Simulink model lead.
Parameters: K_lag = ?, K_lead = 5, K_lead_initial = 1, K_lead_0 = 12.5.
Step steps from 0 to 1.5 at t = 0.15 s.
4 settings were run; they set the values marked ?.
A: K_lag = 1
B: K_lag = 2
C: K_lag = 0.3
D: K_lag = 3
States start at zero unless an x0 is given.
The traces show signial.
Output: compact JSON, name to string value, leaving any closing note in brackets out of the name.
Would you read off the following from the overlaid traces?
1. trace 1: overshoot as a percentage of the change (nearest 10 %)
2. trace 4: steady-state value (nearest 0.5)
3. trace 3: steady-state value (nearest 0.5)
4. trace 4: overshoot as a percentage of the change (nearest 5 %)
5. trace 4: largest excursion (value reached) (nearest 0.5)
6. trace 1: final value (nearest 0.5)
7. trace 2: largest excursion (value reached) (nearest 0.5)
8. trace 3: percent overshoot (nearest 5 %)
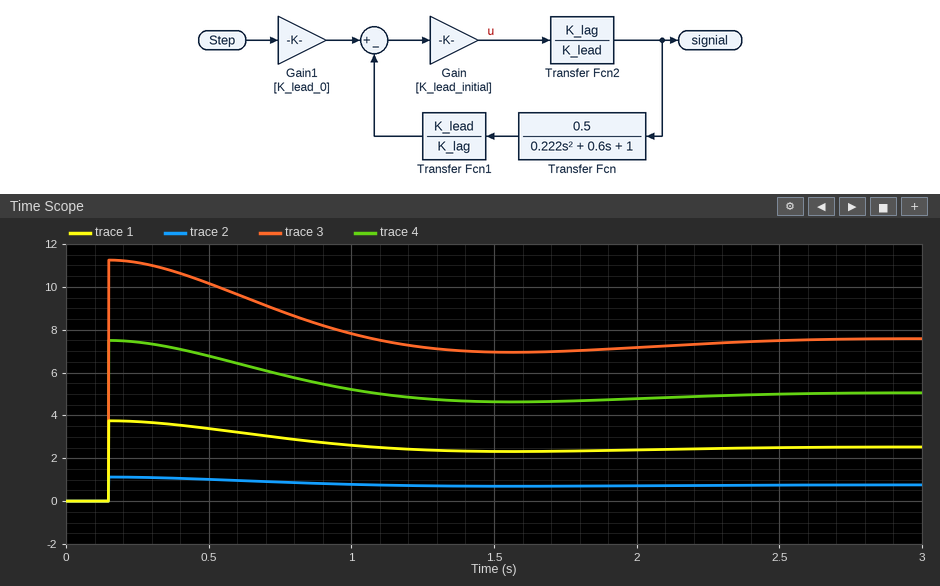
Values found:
{"trace 1: overshoot as a percentage of the change": "50 %", "trace 4: steady-state value": "5.0", "trace 3: steady-state value": "7.5", "trace 4: overshoot as a percentage of the change": "50 %", "trace 4: largest excursion (value reached)": "7.5", "trace 1: final value": "2.5", "trace 2: largest excursion (value reached)": "1.0", "trace 3: percent overshoot": "50 %"}
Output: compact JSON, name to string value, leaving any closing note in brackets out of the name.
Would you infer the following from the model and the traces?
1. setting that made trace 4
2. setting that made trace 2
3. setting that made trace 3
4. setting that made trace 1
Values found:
{"setting that made trace 4": "B", "setting that made trace 2": "C", "setting that made trace 3": "D", "setting that made trace 1": "A"}
